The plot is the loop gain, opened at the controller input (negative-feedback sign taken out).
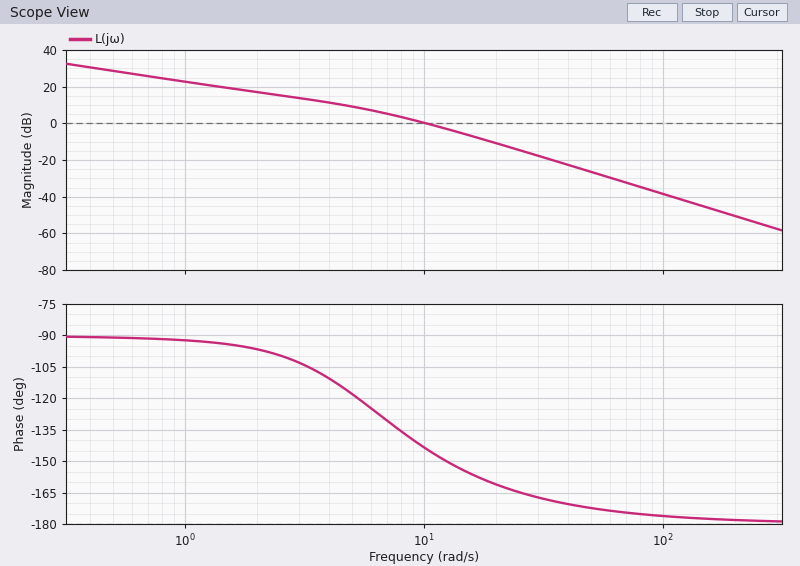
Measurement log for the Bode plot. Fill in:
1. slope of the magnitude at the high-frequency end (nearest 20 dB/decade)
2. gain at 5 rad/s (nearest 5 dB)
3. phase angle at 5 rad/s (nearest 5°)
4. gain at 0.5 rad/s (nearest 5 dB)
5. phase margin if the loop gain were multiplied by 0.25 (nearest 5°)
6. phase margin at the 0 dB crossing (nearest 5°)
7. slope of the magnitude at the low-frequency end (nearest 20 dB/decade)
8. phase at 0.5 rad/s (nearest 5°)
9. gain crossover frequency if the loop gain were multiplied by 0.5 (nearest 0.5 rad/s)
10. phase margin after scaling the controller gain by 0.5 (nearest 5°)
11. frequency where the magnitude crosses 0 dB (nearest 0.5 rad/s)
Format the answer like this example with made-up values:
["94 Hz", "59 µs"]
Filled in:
["-40 dB/decade", "10 dB", "-120°", "30 dB", "70°", "35°", "-20 dB/decade", "-90°", "6.5 rad/s", "50°", "10.0 rad/s"]
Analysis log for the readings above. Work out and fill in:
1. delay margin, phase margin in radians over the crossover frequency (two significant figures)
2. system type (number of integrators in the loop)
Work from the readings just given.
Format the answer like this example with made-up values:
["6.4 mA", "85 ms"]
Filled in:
["0.061 s", "1"]
